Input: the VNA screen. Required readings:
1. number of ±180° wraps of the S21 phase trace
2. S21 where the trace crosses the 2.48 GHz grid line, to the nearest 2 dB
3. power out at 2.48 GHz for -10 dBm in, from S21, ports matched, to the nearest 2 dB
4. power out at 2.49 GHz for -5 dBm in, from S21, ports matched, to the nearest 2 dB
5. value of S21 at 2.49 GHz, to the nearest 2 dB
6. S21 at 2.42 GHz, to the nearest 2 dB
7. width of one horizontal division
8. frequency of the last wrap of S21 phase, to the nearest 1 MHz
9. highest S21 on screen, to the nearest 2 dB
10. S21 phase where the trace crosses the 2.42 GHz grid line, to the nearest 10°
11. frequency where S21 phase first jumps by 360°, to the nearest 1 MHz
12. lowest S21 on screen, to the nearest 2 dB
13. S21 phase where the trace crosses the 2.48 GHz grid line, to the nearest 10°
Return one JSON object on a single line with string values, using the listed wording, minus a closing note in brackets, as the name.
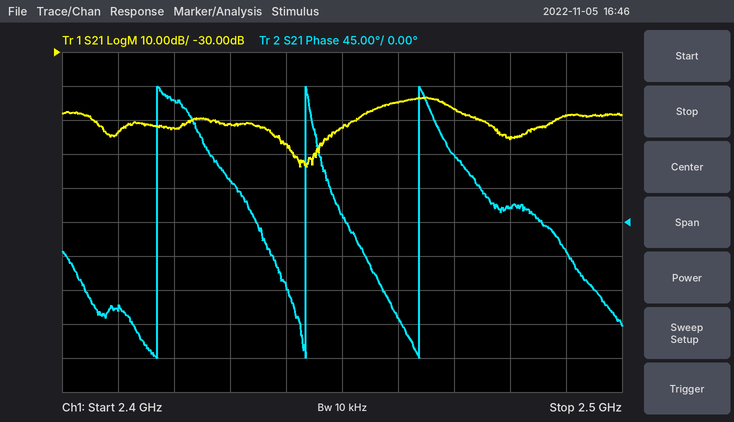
{"number of ±180° wraps of the S21 phase trace": "3", "S21 where the trace crosses the 2.48 GHz grid line, to the nearest 2 dB": "-56 dB", "power out at 2.48 GHz for -10 dBm in, from S21, ports matched, to the nearest 2 dB": "-66 dBm", "power out at 2.49 GHz for -5 dBm in, from S21, ports matched, to the nearest 2 dB": "-54 dBm", "value of S21 at 2.49 GHz, to the nearest 2 dB": "-48 dB", "S21 at 2.42 GHz, to the nearest 2 dB": "-52 dB", "width of one horizontal division": "10 MHz", "frequency of the last wrap of S21 phase, to the nearest 1 MHz": "2.464 GHz", "highest S21 on screen, to the nearest 2 dB": "-44 dB", "S21 phase where the trace crosses the 2.42 GHz grid line, to the nearest 10°": "160°", "frequency where S21 phase first jumps by 360°, to the nearest 1 MHz": "2.417 GHz", "lowest S21 on screen, to the nearest 2 dB": "-64 dB", "S21 phase where the trace crosses the 2.48 GHz grid line, to the nearest 10°": "20°"}
